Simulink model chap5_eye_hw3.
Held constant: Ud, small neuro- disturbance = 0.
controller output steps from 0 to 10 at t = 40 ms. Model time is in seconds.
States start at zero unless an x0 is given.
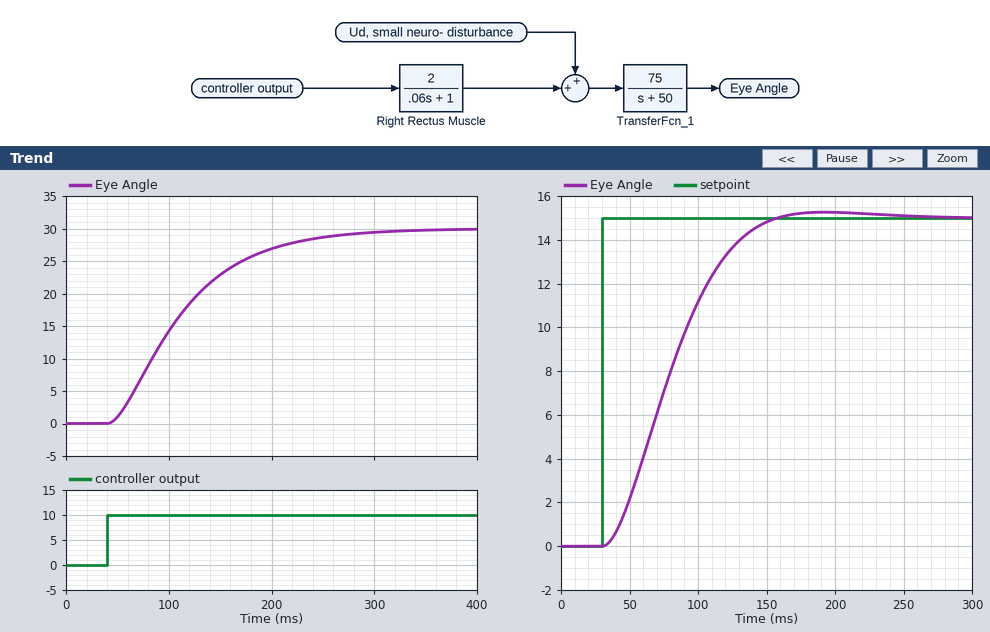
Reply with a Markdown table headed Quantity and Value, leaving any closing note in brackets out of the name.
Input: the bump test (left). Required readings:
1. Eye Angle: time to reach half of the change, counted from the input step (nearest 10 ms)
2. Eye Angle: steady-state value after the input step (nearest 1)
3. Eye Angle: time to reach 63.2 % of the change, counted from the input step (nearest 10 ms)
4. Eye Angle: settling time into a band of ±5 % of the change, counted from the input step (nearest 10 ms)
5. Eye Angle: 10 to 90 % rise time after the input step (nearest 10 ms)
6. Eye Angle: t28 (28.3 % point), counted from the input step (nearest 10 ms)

| Quantity | Value |
|---|---|
| Eye Angle: time to reach half of the change, counted from the input step | 60 ms |
| Eye Angle: steady-state value after the input step | 30 |
| Eye Angle: time to reach 63.2 % of the change, counted from the input step | 80 ms |
| Eye Angle: settling time into a band of ±5 % of the change, counted from the input step | 200 ms |
| Eye Angle: 10 to 90 % rise time after the input step | 140 ms |
| Eye Angle: t28 (28.3 % point), counted from the input step | 40 ms |
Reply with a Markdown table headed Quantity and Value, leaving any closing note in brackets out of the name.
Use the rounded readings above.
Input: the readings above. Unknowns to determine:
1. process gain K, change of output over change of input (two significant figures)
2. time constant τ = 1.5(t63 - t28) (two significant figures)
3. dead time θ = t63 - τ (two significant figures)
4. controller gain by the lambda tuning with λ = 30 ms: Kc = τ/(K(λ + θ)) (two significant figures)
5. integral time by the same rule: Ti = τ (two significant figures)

| Quantity | Value |
|---|---|
| process gain K, change of output over change of input | 3.0 |
| time constant τ = 1.5(t63 - t28) | 60 ms |
| dead time θ = t63 - τ | 20 ms |
| controller gain by the lambda tuning with λ = 30 ms: Kc = τ/(K(λ + θ)) | 0.40 |
| integral time by the same rule: Ti = τ | 60 ms |
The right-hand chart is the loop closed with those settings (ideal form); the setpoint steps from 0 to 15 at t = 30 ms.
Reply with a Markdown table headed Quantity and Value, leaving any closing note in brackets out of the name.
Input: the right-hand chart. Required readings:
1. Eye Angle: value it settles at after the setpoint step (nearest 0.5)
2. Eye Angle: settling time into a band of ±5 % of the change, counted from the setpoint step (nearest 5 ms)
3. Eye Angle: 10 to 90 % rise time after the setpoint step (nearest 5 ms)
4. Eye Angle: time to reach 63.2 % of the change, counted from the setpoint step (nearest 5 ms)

| Quantity | Value |
|---|---|
| Eye Angle: value it settles at after the setpoint step | 15.0 |
| Eye Angle: settling time into a band of ±5 % of the change, counted from the setpoint step | 105 ms |
| Eye Angle: 10 to 90 % rise time after the setpoint step | 75 ms |
| Eye Angle: time to reach 63.2 % of the change, counted from the setpoint step | 60 ms |
